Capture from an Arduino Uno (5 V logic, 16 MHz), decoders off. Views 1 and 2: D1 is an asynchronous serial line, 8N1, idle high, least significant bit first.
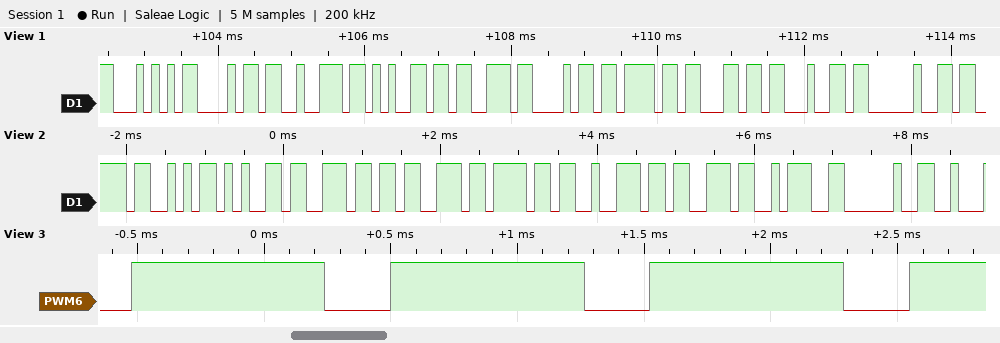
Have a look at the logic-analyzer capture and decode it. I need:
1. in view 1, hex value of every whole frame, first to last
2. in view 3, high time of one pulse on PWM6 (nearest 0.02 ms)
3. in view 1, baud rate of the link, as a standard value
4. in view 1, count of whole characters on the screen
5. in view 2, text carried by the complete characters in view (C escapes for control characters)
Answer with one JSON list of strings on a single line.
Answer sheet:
["54 68 72 65 73 68 6F 6C 64 20", "0.76 ms", "9600 baud", "10", "\"Sensors: \""]
